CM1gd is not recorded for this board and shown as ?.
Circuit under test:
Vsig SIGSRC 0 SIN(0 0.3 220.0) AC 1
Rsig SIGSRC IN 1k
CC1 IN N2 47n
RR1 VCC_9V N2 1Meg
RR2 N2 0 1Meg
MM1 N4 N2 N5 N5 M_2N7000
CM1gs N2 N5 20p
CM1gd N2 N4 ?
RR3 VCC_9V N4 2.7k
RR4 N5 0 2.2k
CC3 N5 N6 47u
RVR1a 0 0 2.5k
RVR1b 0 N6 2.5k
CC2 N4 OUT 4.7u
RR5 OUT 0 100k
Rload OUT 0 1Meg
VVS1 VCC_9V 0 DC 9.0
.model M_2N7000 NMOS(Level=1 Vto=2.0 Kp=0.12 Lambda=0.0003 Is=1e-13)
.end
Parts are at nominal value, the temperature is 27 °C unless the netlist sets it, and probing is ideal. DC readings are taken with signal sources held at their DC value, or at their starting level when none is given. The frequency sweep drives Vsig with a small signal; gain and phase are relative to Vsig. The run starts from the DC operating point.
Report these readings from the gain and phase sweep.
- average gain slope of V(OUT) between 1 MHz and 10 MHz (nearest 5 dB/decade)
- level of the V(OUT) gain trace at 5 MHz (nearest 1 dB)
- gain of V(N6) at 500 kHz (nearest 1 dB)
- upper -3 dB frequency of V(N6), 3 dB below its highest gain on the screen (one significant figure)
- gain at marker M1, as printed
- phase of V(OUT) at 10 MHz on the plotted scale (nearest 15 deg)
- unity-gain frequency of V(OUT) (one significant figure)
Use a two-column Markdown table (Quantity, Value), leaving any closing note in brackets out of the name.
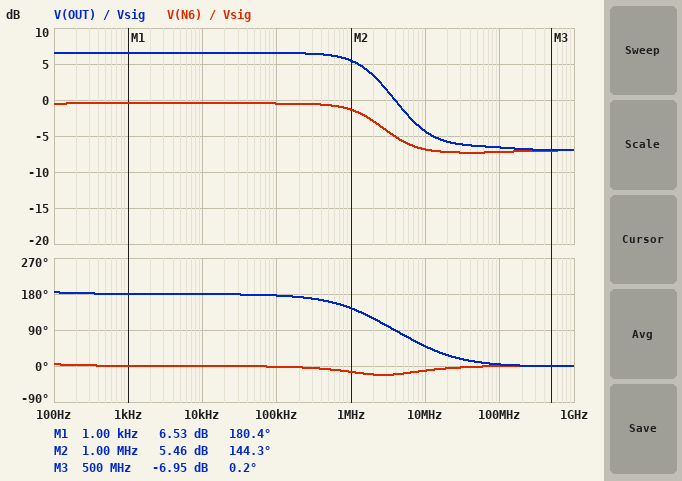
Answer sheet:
| Quantity | Value |
|---|---|
| average gain slope of V(OUT) between 1 MHz and 10 MHz | -10 dB/decade |
| level of the V(OUT) gain trace at 5 MHz | -1 dB |
| gain of V(N6) at 500 kHz | -1 dB |
| upper -3 dB frequency of V(N6), 3 dB below its highest gain on the screen | 2 MHz |
| gain at marker M1, as printed | 6.53 dB |
| phase of V(OUT) at 10 MHz on the plotted scale | 45 deg |
| unity-gain frequency of V(OUT) | 4 MHz |
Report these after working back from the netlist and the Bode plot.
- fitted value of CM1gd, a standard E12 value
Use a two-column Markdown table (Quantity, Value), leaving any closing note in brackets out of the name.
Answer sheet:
| Quantity | Value |
|---|---|
| fitted value of CM1gd, a standard E12 value | 15 pF |
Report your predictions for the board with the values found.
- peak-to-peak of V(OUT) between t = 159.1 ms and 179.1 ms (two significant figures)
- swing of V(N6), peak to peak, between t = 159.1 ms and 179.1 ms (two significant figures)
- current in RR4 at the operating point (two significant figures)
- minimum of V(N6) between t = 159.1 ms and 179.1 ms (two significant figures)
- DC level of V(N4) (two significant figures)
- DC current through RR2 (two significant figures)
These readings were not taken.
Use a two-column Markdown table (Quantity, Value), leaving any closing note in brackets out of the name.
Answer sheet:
| Quantity | Value |
|---|---|
| peak-to-peak of V(OUT) between t = 159.1 ms and 179.1 ms | 1.3 V |
| swing of V(N6), peak to peak, between t = 159.1 ms and 179.1 ms | 570 mV |
| current in RR4 at the operating point | 1.1 mA |
| minimum of V(N6) between t = 159.1 ms and 179.1 ms | -280 mV |
| DC level of V(N4) | 6.1 V |
| DC current through RR2 | 4.5 µA |
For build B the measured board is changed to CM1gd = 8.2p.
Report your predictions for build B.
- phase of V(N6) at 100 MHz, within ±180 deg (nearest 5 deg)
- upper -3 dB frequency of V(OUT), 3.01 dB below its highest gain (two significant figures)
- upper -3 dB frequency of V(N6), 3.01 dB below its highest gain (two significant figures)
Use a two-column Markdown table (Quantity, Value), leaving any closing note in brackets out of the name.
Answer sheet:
| Quantity | Value |
|---|---|
| phase of V(N6) at 100 MHz, within ±180 deg | 0 deg |
| upper -3 dB frequency of V(OUT), 3.01 dB below its highest gain | 3.5 MHz |
| upper -3 dB frequency of V(N6), 3.01 dB below its highest gain | 4.3 MHz |
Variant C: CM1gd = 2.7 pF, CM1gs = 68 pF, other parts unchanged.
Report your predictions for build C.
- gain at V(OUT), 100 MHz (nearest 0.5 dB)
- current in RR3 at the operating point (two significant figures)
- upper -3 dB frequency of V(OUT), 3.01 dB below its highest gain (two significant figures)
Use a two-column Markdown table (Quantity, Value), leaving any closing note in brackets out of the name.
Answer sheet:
| Quantity | Value |
|---|---|
| gain at V(OUT), 100 MHz | -6.0 dB |
| current in RR3 at the operating point | 1.1 mA |
| upper -3 dB frequency of V(OUT), 3.01 dB below its highest gain | 8.7 MHz |
